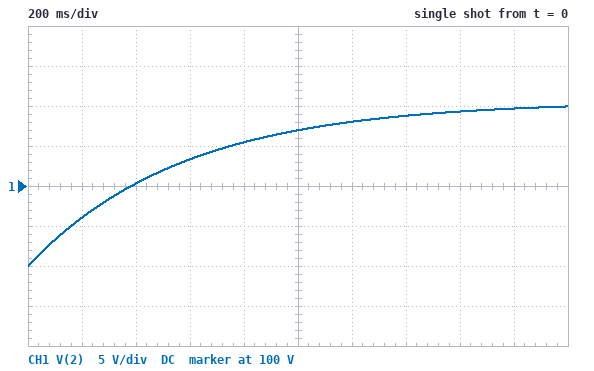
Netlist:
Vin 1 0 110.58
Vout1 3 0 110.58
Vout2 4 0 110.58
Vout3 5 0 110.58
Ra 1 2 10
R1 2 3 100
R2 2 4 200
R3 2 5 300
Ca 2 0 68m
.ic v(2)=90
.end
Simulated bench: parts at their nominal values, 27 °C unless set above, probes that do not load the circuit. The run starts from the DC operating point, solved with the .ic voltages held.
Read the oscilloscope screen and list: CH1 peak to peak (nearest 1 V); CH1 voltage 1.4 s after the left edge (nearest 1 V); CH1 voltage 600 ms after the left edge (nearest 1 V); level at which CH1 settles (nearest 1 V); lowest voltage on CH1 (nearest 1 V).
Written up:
20 V
109 V
103 V
110 V
90 V
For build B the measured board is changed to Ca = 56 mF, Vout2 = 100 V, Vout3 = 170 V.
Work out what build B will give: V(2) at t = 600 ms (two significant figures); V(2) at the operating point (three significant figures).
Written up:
110 V
112 V
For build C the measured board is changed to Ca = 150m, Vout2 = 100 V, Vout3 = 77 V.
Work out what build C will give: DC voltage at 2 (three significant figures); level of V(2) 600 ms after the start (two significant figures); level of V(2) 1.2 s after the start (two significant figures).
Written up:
109 V
97 V
100 V
